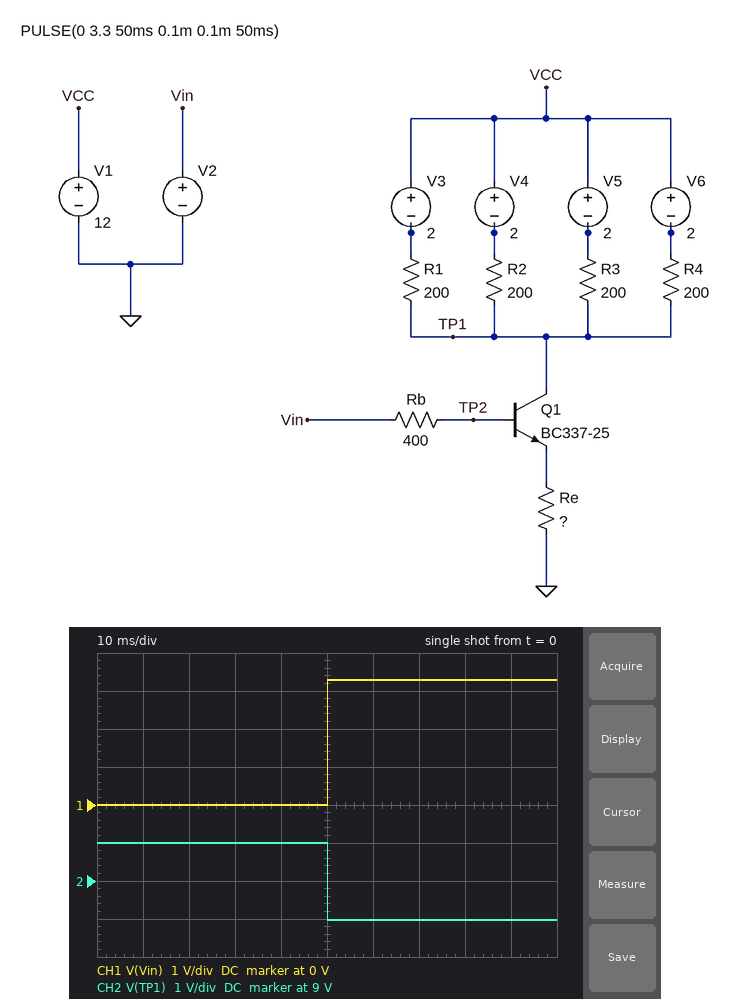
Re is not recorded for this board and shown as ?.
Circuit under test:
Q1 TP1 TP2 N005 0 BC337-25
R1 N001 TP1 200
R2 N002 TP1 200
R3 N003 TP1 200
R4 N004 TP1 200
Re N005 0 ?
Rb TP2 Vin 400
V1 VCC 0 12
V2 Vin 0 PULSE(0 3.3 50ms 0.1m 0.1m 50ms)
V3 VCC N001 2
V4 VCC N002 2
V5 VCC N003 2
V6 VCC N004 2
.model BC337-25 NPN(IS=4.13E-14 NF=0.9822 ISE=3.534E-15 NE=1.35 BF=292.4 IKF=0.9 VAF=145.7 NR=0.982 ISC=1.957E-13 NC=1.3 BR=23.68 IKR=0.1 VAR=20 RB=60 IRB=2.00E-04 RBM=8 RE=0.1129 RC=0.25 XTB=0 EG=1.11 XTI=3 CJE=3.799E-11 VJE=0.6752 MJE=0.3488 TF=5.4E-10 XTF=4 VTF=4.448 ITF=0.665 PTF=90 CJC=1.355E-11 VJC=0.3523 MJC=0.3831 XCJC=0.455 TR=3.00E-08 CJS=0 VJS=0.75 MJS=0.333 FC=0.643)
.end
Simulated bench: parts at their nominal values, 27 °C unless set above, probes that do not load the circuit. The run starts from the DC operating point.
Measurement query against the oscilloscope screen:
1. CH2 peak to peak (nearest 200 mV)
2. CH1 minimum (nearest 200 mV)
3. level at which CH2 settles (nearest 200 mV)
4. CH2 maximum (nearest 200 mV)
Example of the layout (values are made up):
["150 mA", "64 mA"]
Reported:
["2.0 V", "0 V", "8.0 V", "10.0 V"]
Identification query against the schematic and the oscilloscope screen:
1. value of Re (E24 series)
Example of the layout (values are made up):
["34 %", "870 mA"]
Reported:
["62 Ω"]
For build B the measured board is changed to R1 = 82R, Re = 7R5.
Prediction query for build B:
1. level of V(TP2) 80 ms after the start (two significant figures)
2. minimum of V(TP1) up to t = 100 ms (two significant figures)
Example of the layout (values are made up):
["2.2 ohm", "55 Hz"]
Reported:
["2.5 V", "1.8 V"]
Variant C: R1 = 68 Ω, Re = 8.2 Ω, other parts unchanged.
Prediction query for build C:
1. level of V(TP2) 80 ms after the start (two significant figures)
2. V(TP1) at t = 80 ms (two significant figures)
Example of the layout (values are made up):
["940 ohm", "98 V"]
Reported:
["2.7 V", "2.1 V"]
